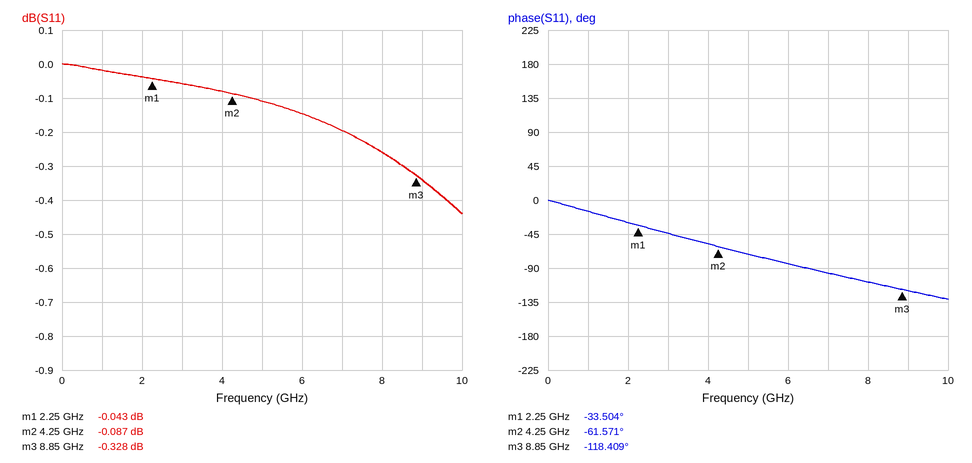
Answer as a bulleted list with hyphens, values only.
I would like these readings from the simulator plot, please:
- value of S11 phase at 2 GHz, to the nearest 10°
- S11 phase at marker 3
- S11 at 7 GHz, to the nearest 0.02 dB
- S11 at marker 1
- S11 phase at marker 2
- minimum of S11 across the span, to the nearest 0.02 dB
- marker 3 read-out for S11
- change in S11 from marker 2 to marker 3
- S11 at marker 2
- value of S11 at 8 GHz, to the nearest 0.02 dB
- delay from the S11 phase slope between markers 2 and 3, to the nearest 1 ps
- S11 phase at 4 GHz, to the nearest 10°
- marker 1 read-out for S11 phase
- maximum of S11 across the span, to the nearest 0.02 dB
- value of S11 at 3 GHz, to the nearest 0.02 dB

- -30°
- -118.409°
- -0.20 dB
- -0.043 dB
- -61.571°
- -0.44 dB
- -0.328 dB
- -0.241 dB
- -0.087 dB
- -0.26 dB
- 34 ps
- -60°
- -33.504°
- 0.00 dB
- -0.06 dB
